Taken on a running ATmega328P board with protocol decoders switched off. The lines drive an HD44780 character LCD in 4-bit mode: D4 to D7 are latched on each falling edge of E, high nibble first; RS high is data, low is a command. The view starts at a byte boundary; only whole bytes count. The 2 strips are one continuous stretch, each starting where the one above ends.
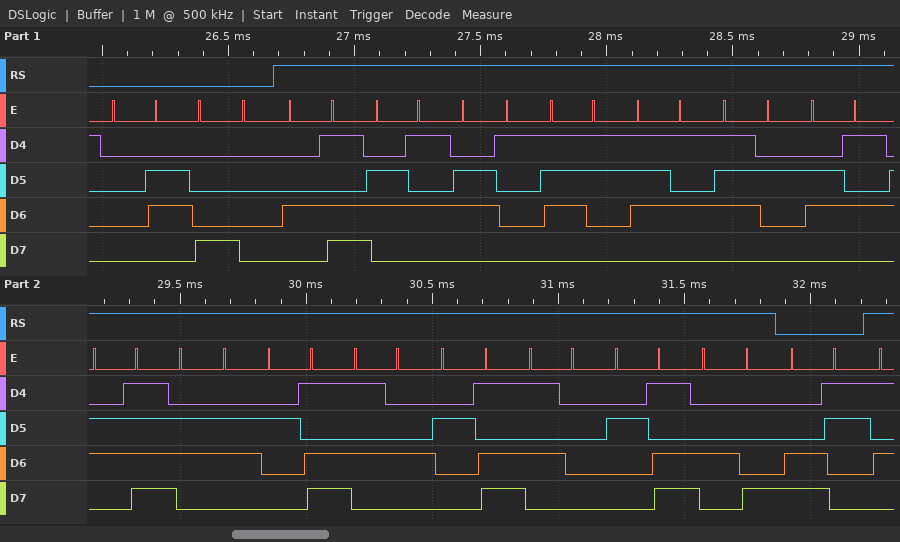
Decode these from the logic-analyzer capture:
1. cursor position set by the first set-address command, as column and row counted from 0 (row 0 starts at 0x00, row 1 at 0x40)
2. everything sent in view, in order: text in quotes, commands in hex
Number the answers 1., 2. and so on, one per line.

1. column 0, row 0
2. 0x06 0x80 "Measureof-T-P-H" 0xC3
